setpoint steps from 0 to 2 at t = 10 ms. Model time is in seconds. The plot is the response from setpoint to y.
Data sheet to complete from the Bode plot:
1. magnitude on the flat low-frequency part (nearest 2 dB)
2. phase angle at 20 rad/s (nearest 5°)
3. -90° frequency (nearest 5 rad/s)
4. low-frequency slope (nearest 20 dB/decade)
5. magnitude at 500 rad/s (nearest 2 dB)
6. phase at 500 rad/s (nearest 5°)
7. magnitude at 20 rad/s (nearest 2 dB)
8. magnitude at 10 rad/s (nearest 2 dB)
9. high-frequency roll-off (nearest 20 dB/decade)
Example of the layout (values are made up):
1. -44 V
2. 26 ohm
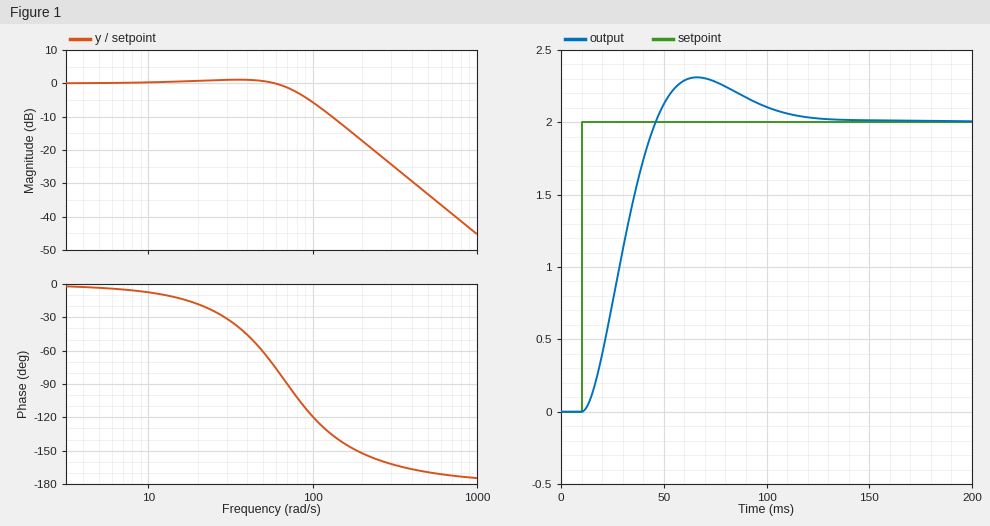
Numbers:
1. 0 dB
2. -20°
3. 70 rad/s
4. 0 dB/decade
5. -34 dB
6. -170°
7. 0 dB
8. 0 dB
9. -40 dB/decade
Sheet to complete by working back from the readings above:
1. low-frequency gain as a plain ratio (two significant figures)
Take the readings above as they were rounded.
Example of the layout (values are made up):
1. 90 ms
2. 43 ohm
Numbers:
1. 1.0
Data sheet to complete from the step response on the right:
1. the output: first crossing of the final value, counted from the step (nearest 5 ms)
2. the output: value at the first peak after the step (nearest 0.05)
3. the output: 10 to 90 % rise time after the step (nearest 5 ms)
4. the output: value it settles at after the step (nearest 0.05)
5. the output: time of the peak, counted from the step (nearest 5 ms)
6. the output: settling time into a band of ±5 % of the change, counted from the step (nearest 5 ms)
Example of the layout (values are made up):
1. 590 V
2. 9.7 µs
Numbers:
1. 35 ms
2. 2.30
3. 25 ms
4. 2.00
5. 55 ms
6. 90 ms
